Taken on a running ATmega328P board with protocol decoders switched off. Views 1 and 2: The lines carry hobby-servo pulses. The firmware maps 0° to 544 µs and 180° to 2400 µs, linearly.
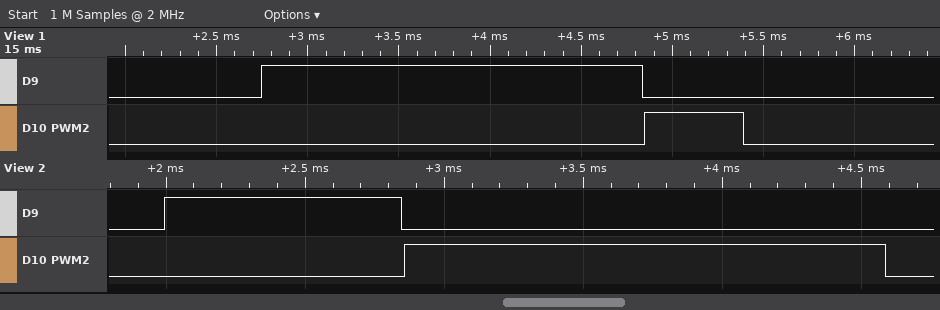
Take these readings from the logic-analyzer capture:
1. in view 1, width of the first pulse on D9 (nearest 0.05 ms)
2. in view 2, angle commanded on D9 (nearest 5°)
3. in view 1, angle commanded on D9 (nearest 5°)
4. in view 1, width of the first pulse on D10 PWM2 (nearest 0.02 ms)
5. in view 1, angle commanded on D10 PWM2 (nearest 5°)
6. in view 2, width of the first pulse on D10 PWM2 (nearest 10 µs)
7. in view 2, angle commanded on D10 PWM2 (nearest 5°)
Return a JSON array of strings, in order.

["2.10 ms", "30°", "150°", "0.54 ms", "0°", "1730 µs", "115°"]
